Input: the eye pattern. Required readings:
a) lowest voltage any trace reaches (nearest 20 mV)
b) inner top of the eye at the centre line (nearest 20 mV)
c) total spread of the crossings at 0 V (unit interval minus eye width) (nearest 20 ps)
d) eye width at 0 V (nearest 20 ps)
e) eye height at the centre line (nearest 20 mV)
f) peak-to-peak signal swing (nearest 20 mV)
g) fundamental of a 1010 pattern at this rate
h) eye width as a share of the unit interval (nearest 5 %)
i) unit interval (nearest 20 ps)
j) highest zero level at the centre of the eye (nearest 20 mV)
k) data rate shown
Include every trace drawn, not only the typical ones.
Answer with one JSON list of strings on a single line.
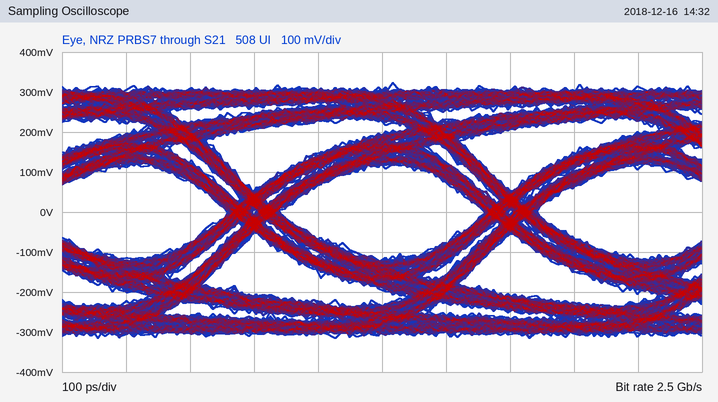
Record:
["-320 mV", "120 mV", "80 ps", "320 ps", "240 mV", "640 mV", "1.25 GHz", "80 %", "400 ps", "-120 mV", "2.5 Gb/s"]
